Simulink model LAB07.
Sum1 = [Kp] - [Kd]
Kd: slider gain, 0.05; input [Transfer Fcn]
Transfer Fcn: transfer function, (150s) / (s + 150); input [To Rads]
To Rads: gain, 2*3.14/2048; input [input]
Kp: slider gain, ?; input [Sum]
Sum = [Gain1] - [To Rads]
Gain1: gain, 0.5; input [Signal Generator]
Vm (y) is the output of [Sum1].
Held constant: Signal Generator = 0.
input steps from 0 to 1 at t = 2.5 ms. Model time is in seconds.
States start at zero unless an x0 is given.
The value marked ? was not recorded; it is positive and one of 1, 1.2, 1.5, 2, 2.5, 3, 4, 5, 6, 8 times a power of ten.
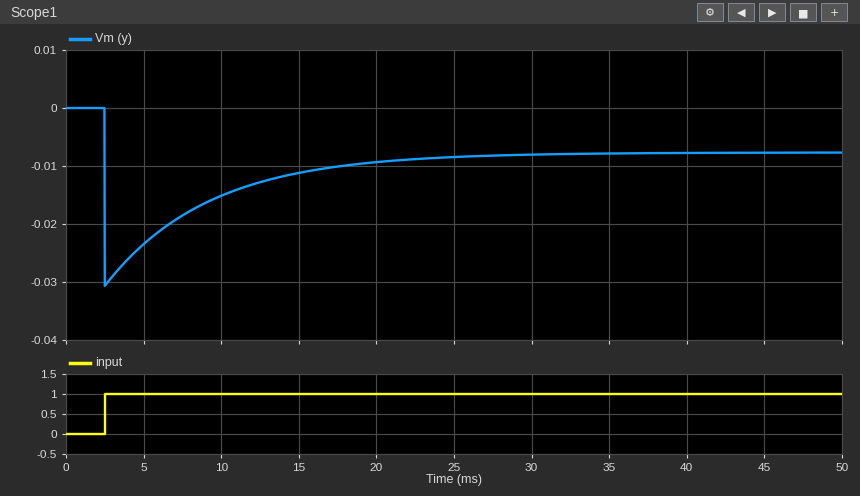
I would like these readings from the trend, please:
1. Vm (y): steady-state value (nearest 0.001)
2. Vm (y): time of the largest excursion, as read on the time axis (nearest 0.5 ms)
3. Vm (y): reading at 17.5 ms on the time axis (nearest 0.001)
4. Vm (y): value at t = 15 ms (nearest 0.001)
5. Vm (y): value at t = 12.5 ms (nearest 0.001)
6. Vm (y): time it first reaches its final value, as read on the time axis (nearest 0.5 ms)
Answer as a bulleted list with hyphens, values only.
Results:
- -0.008
- 2.5 ms
- -0.010
- -0.011
- -0.013
- 2.5 ms
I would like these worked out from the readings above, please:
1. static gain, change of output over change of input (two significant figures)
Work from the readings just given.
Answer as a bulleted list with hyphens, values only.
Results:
- -0.0080
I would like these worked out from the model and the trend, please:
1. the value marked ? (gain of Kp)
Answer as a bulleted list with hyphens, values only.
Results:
- 2.5
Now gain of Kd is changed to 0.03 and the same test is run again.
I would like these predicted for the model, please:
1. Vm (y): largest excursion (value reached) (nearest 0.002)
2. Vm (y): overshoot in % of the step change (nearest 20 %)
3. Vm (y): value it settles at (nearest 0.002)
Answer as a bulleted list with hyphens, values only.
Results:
- -0.022
- 180 %
- -0.008
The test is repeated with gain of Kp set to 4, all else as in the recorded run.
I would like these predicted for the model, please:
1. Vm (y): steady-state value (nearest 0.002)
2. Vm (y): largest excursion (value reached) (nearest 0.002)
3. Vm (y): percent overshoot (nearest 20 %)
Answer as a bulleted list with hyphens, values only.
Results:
- -0.012
- -0.036
- 180 %
